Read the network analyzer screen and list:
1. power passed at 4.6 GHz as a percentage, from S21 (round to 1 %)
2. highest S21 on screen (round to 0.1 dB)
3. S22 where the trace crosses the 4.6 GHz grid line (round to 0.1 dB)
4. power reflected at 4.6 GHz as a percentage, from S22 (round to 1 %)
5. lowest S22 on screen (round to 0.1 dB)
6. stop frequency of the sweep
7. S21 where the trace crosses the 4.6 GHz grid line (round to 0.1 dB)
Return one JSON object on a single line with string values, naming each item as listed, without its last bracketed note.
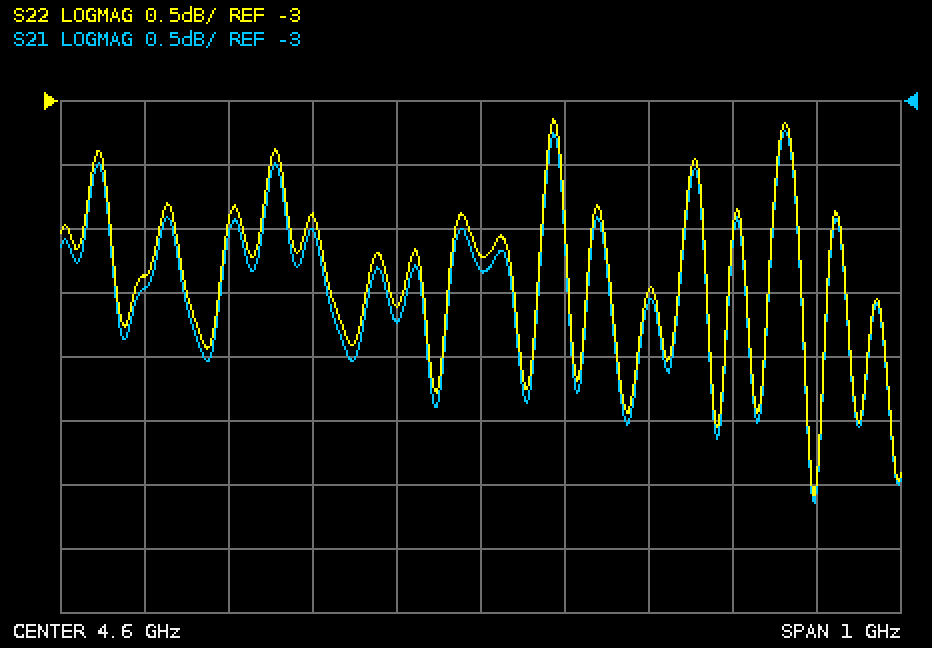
{"power passed at 4.6 GHz as a percentage, from S21": "37 %", "highest S21 on screen": "-3.2 dB", "S22 where the trace crosses the 4.6 GHz grid line": "-4.2 dB", "power reflected at 4.6 GHz as a percentage, from S22": "38 %", "lowest S22 on screen": "-6.1 dB", "stop frequency of the sweep": "5.1 GHz", "S21 where the trace crosses the 4.6 GHz grid line": "-4.3 dB"}
